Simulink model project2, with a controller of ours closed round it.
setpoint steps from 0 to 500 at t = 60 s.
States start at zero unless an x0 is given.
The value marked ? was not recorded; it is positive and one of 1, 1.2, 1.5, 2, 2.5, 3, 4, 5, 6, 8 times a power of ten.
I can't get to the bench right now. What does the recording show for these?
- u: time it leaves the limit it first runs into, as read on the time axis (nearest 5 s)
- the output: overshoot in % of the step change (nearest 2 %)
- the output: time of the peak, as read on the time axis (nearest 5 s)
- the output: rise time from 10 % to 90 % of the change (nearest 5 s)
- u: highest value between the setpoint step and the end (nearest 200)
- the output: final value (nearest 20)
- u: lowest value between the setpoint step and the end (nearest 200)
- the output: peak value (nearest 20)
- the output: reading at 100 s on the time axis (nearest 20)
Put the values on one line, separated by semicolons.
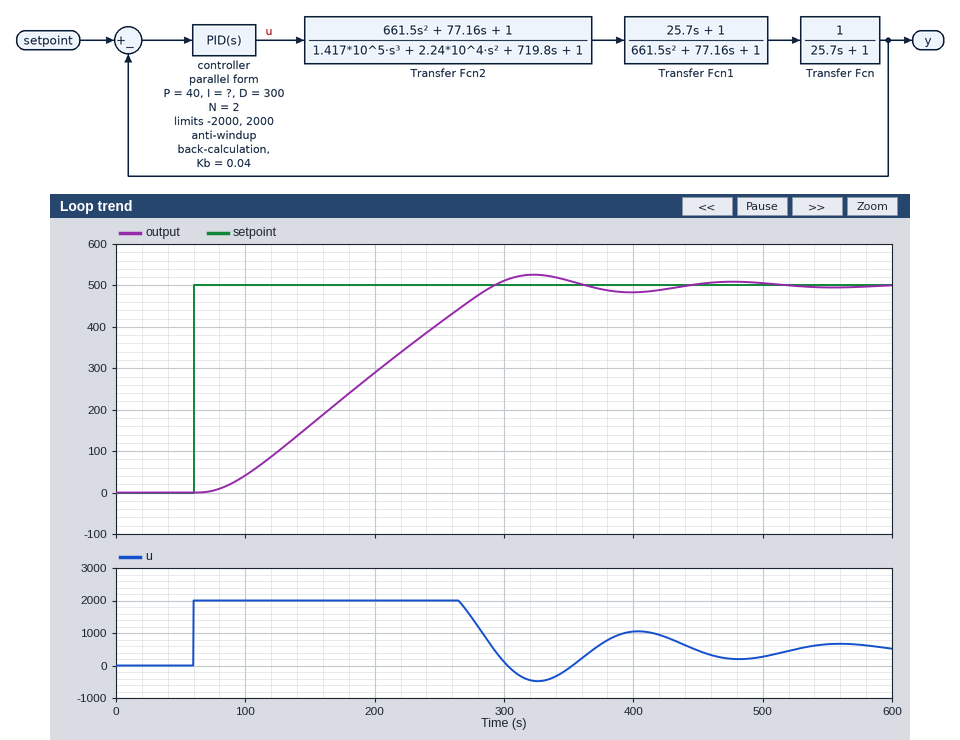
265 s; 6 %; 325 s; 165 s; 2000; 500; -400; 520; 40
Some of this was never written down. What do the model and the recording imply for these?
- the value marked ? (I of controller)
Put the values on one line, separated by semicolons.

0.8
